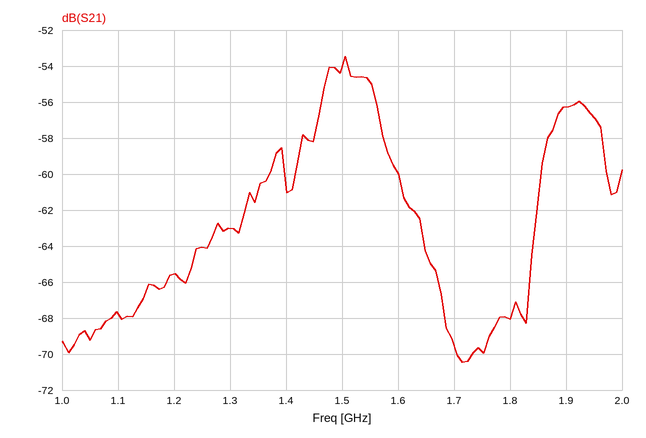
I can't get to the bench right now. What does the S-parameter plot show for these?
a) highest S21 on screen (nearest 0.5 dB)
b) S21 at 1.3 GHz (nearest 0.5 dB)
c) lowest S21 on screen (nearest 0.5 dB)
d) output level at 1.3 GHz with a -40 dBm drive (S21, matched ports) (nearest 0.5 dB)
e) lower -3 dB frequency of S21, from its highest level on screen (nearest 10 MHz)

-53.5 dB
-63.0 dB
-70.5 dB
-103.0 dBm
1.46 GHz
